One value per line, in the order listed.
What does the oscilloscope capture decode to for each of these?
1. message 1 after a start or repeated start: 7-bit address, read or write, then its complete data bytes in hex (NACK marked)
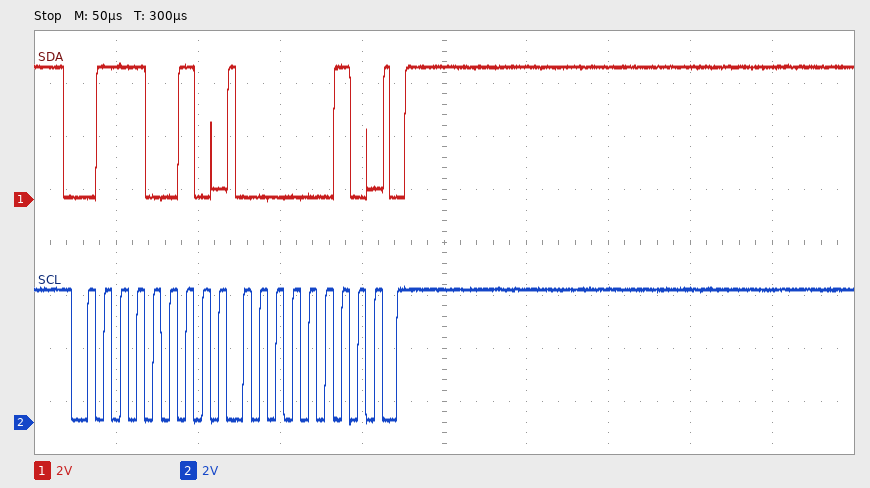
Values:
0x39 write: 02
